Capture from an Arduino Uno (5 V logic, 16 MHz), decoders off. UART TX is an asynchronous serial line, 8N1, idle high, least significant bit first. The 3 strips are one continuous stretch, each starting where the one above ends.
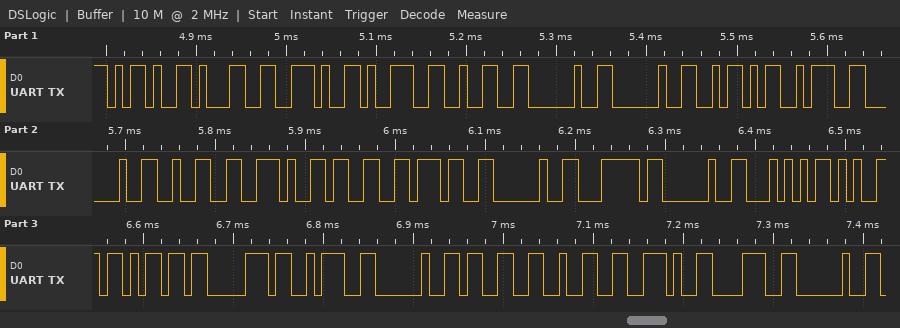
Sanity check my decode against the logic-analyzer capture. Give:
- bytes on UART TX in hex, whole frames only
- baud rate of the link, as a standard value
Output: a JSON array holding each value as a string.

["2D 31 2E 39 32 20 20 5A 3A 20 32 2E 33 37 20 7C 20 54 65 6D 70 3A 20 33 32 2E 38 20", "115200 baud"]
